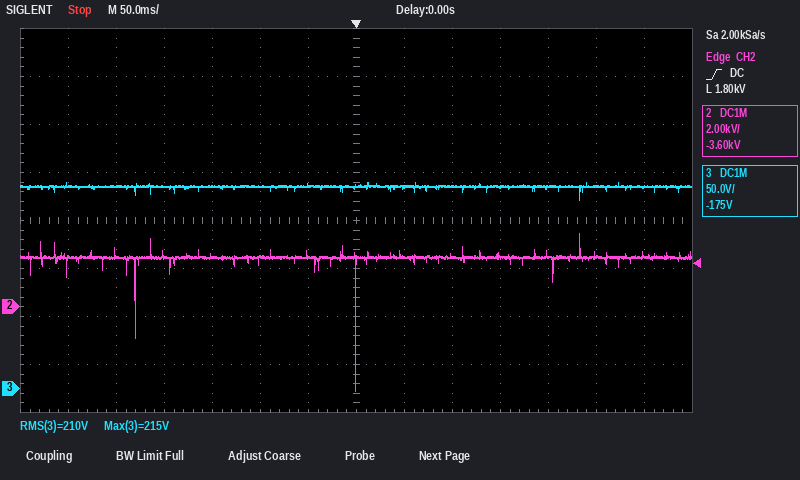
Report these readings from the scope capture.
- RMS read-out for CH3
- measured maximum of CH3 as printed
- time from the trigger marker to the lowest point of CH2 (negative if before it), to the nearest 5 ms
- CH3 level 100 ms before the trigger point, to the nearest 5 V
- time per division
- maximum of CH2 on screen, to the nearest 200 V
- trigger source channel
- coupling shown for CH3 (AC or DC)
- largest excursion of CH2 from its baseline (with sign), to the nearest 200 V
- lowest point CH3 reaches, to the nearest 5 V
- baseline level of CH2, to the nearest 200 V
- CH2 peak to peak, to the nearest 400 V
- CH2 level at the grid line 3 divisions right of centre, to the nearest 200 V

210 V
215 V
0 ms
210 V
50 ms
3.0 kV
CH2
DC
-5.6 kV
195 V
2.0 kV
6.4 kV
2.2 kV
